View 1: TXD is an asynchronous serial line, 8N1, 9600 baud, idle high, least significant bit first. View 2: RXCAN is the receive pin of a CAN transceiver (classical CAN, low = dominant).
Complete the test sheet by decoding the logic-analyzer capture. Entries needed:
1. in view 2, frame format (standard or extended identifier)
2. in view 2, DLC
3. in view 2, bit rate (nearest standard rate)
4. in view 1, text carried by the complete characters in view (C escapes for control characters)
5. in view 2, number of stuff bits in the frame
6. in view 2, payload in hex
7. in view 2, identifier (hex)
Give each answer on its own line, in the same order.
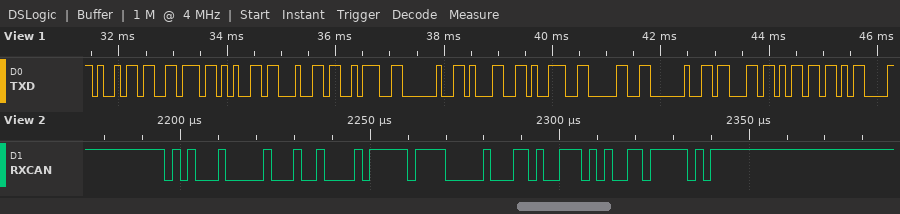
standard
4
500 kbit/s
"ived: 190 cm\r"
4
85 FF 00 D3
0x510
